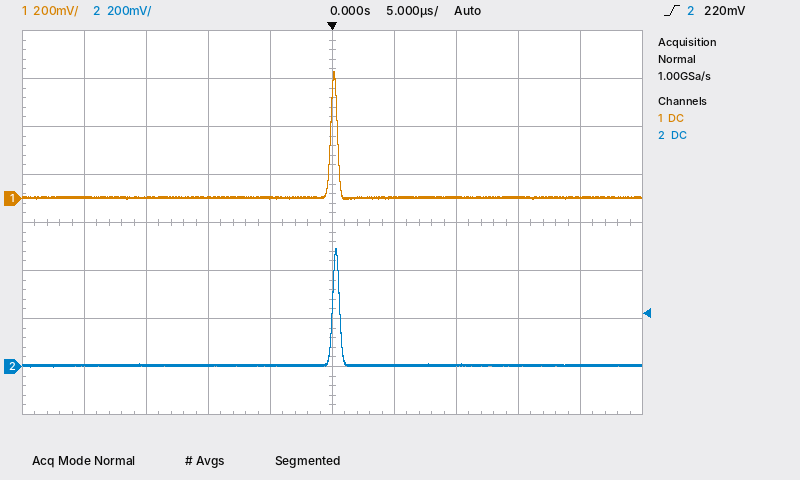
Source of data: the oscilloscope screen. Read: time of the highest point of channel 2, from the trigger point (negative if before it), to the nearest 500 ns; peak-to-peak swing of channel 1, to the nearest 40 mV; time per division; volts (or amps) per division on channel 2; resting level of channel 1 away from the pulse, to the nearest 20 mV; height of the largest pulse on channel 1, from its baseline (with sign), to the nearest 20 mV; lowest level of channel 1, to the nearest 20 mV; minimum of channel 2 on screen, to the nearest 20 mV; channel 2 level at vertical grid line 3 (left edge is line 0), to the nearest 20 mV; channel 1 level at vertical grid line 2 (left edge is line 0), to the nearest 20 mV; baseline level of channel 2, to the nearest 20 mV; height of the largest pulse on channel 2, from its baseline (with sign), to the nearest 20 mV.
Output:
+500 ns
520 mV
5 µs
200 mV
0 mV
+520 mV
0 mV
0 mV
0 mV
0 mV
0 mV
+480 mV
